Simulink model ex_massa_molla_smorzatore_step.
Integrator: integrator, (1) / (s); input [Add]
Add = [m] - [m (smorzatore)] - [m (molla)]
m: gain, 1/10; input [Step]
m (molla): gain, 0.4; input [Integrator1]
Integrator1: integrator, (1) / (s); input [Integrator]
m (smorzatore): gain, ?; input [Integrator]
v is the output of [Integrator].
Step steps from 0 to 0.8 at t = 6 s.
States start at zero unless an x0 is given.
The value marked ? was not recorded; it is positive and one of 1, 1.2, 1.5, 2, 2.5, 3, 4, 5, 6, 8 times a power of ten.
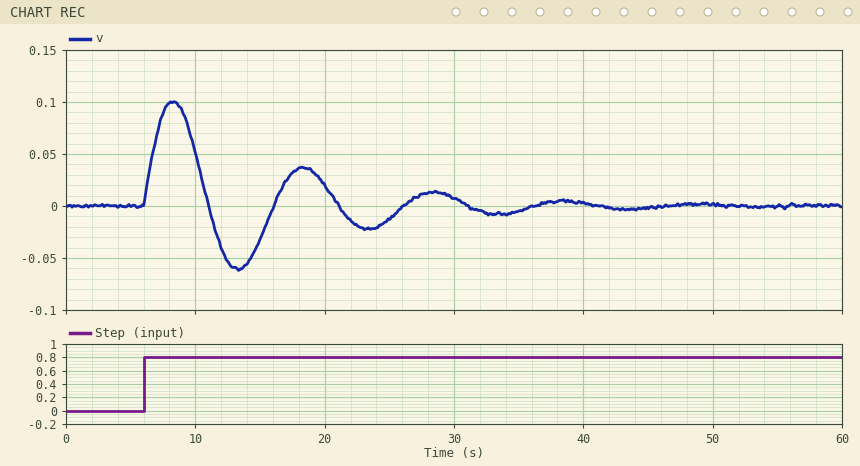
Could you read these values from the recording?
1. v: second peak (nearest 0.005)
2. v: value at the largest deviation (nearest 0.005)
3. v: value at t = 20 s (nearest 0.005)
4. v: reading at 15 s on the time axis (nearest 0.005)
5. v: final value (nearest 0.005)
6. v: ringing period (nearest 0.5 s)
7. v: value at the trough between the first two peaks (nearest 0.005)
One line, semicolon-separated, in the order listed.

0.035; 0.100; 0.020; -0.030; 0.000; 10.0 s; -0.060
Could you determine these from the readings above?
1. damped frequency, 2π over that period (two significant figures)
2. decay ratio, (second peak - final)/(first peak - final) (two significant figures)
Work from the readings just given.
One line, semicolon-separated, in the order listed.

0.63 rad/s; 0.35
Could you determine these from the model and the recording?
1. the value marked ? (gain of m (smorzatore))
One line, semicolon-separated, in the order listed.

0.2
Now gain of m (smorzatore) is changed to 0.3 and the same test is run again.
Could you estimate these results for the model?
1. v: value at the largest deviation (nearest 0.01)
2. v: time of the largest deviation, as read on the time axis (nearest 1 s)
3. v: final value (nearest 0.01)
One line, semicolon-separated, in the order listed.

0.09; 8 s; 0.00
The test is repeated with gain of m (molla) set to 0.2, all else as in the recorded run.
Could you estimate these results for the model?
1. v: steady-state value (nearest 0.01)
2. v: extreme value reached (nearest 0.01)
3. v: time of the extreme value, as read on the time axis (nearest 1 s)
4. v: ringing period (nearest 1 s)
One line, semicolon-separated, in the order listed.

0.00; 0.13; 9 s; 14 s
